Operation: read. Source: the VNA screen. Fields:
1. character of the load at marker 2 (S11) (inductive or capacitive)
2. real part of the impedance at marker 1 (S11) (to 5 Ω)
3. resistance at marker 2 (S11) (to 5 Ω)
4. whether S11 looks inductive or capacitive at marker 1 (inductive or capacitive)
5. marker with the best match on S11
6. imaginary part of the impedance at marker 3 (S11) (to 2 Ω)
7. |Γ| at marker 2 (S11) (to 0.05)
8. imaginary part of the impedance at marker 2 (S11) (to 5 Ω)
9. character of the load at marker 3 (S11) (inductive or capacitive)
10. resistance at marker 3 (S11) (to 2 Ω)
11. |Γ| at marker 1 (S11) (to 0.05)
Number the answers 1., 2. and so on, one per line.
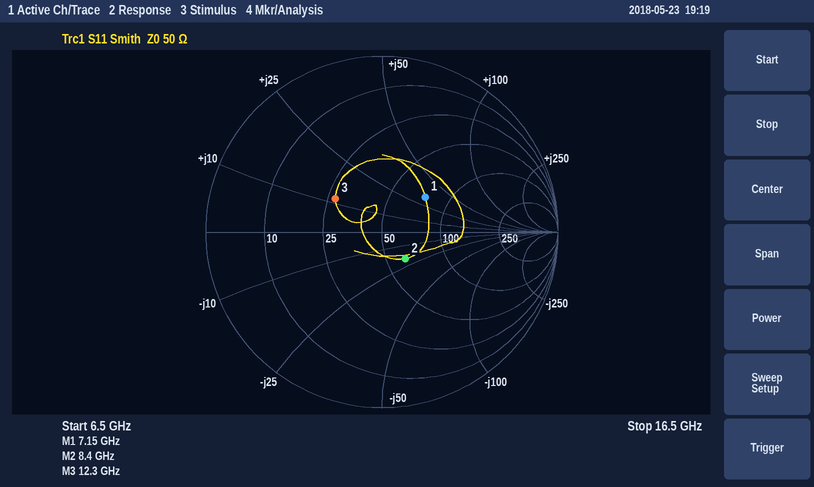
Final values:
1. capacitive
2. 75 Ω
3. 60 Ω
4. inductive
5. marker 2
6. +12 Ω
7. 0.20
8. -20 Ω
9. inductive
10. 28 Ω
11. 0.30
